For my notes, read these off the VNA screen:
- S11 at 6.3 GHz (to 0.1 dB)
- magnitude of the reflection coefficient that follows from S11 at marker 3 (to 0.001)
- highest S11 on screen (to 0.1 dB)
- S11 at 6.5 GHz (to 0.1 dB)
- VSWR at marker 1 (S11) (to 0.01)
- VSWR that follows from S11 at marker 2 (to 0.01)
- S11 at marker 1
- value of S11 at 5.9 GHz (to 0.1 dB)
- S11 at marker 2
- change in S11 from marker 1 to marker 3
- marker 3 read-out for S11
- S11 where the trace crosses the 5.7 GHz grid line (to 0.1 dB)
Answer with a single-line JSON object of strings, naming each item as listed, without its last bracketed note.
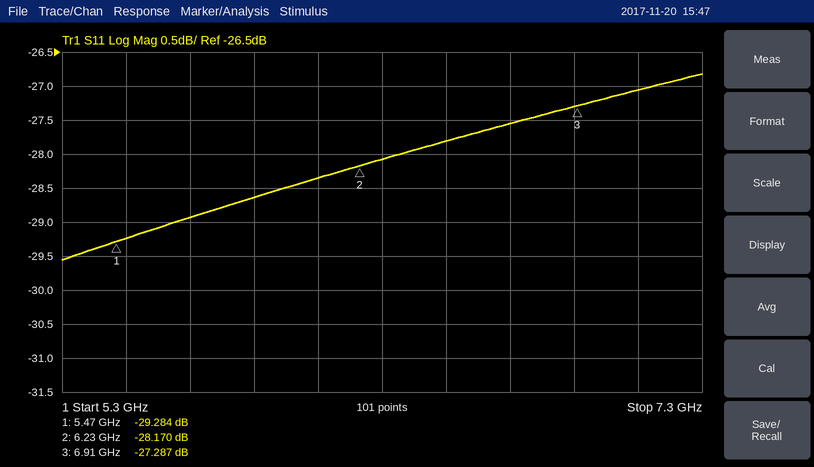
{"S11 at 6.3 GHz": "-28.1 dB", "magnitude of the reflection coefficient that follows from S11 at marker 3": "0.043", "highest S11 on screen": "-26.8 dB", "S11 at 6.5 GHz": "-27.8 dB", "VSWR at marker 1 (S11)": "1.07", "VSWR that follows from S11 at marker 2": "1.08", "S11 at marker 1": "-29.284 dB", "value of S11 at 5.9 GHz": "-28.6 dB", "S11 at marker 2": "-28.170 dB", "change in S11 from marker 1 to marker 3": "1.997 dB", "marker 3 read-out for S11": "-27.287 dB", "S11 where the trace crosses the 5.7 GHz grid line": "-28.9 dB"}
